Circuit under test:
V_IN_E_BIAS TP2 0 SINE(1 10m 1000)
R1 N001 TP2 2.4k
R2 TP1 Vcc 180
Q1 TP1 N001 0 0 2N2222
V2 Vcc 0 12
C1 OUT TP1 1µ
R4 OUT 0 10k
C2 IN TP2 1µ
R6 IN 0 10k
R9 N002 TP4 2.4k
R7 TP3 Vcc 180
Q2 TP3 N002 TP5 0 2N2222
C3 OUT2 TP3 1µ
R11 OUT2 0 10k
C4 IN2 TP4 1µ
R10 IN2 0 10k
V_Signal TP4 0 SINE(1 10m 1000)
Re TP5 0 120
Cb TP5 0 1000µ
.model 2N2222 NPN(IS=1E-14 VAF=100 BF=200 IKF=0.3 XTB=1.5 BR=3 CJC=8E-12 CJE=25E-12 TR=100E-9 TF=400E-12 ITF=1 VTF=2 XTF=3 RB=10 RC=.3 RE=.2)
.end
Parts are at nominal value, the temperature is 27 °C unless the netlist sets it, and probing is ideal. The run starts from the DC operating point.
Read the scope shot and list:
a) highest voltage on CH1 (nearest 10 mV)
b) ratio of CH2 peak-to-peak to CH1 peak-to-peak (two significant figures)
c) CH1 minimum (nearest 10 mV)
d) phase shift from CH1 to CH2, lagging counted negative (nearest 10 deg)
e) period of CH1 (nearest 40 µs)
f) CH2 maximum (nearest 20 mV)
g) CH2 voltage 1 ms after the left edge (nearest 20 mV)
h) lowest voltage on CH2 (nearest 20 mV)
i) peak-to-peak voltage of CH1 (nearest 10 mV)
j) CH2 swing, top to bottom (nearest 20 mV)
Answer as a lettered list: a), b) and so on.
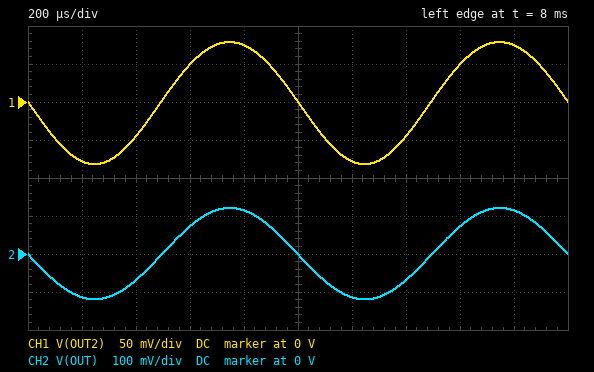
a) 80 mV
b) 1.5
c) -80 mV
d) 0 deg
e) 1.00 ms
f) 120 mV
g) 0 V
h) -120 mV
i) 160 mV
j) 240 mV
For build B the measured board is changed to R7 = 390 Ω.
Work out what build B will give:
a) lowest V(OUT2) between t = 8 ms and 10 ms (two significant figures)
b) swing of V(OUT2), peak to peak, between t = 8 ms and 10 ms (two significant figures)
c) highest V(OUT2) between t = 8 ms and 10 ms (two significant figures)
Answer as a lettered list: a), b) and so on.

a) -170 mV
b) 340 mV
c) 170 mV
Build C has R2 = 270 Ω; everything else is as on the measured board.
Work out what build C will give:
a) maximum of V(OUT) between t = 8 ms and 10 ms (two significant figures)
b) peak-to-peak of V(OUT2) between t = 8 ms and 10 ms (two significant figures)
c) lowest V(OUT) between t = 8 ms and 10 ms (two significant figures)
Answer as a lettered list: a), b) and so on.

a) 170 mV
b) 160 mV
c) -170 mV
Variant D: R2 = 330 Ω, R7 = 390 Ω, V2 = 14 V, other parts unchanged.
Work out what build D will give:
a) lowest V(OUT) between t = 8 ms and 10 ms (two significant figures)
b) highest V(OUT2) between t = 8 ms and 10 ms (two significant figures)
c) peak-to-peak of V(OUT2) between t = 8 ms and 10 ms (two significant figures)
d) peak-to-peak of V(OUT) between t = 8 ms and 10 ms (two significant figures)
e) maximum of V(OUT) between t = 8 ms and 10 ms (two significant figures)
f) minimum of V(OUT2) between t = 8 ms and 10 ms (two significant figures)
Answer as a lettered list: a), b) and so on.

a) -210 mV
b) 170 mV
c) 340 mV
d) 420 mV
e) 210 mV
f) -170 mV
